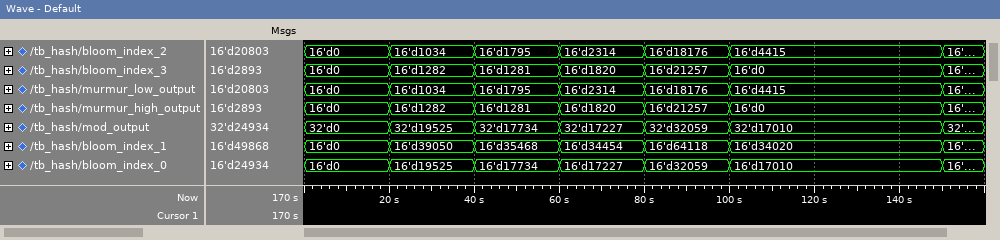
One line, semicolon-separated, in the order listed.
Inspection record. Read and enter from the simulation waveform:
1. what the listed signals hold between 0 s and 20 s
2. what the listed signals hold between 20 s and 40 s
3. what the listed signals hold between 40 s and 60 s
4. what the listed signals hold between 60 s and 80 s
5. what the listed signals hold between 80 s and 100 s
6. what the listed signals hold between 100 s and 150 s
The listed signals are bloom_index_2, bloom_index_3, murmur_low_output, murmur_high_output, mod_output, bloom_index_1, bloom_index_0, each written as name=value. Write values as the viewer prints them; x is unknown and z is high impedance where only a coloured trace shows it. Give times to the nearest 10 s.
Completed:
bloom_index_2=16'd0, bloom_index_3=16'd0, murmur_low_output=16'd0, murmur_high_output=16'd0, mod_output=32'd0, bloom_index_1=16'd0, bloom_index_0=16'd0; bloom_index_2=16'd1034, bloom_index_3=16'd1282, murmur_low_output=16'd1034, murmur_high_output=16'd1282, mod_output=32'd19525, bloom_index_1=16'd39050, bloom_index_0=16'd19525; bloom_index_2=16'd1795, bloom_index_3=16'd1281, murmur_low_output=16'd1795, murmur_high_output=16'd1281, mod_output=32'd17734, bloom_index_1=16'd35468, bloom_index_0=16'd17734; bloom_index_2=16'd2314, bloom_index_3=16'd1820, murmur_low_output=16'd2314, murmur_high_output=16'd1820, mod_output=32'd17227, bloom_index_1=16'd34454, bloom_index_0=16'd17227; bloom_index_2=16'd18176, bloom_index_3=16'd21257, murmur_low_output=16'd18176, murmur_high_output=16'd21257, mod_output=32'd32059, bloom_index_1=16'd64118, bloom_index_0=16'd32059; bloom_index_2=16'd4415, bloom_index_3=16'd0, murmur_low_output=16'd4415, murmur_high_output=16'd0, mod_output=32'd17010, bloom_index_1=16'd34020, bloom_index_0=16'd17010
